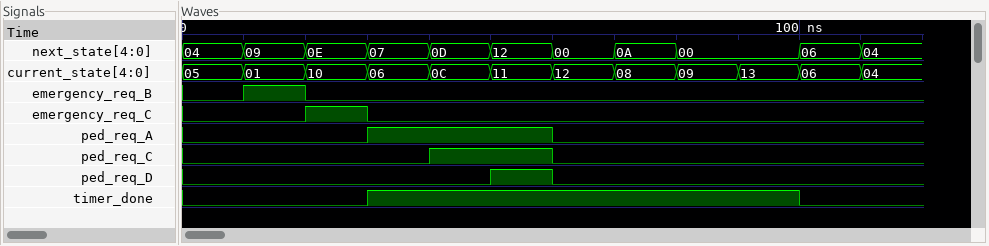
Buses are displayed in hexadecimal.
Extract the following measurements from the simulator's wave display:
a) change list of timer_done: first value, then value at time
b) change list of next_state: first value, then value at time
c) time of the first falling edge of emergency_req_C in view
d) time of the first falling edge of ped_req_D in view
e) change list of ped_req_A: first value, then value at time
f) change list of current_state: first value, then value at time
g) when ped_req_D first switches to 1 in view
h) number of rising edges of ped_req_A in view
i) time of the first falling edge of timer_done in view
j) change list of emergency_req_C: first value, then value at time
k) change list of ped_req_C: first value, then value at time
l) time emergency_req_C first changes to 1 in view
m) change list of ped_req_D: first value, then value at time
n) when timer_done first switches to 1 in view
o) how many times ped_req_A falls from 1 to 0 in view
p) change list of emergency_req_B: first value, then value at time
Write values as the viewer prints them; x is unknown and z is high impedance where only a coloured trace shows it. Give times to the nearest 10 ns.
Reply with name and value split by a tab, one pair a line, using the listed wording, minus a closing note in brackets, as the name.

change list of timer_done: first value, then value at time	0, 1 at 30 ns, 0 at 100 ns
change list of next_state: first value, then value at time	04, 09 at 10 ns, 0E at 20 ns, 07 at 30 ns, 0D at 40 ns, 12 at 50 ns, 00 at 60 ns, 0A at 70 ns, 00 at 80 ns, 06 at 100 ns, 04 at 110 ns
time of the first falling edge of emergency_req_C in view	30 ns
time of the first falling edge of ped_req_D in view	60 ns
change list of ped_req_A: first value, then value at time	0, 1 at 30 ns, 0 at 60 ns
change list of current_state: first value, then value at time	05, 01 at 10 ns, 10 at 20 ns, 06 at 30 ns, 0C at 40 ns, 11 at 50 ns, 12 at 60 ns, 08 at 70 ns, 09 at 80 ns, 13 at 90 ns, 06 at 100 ns, 04 at 110 ns
when ped_req_D first switches to 1 in view	50 ns
number of rising edges of ped_req_A in view	1
time of the first falling edge of timer_done in view	100 ns
change list of emergency_req_C: first value, then value at time	0, 1 at 20 ns, 0 at 30 ns
change list of ped_req_C: first value, then value at time	0, 1 at 40 ns, 0 at 60 ns
time emergency_req_C first changes to 1 in view	20 ns
change list of ped_req_D: first value, then value at time	0, 1 at 50 ns, 0 at 60 ns
when timer_done first switches to 1 in view	30 ns
how many times ped_req_A falls from 1 to 0 in view	1
change list of emergency_req_B: first value, then value at time	0, 1 at 10 ns, 0 at 20 ns
